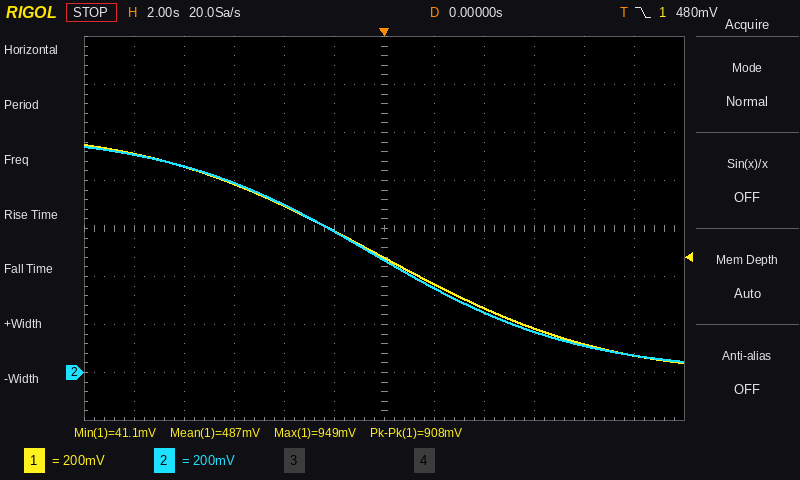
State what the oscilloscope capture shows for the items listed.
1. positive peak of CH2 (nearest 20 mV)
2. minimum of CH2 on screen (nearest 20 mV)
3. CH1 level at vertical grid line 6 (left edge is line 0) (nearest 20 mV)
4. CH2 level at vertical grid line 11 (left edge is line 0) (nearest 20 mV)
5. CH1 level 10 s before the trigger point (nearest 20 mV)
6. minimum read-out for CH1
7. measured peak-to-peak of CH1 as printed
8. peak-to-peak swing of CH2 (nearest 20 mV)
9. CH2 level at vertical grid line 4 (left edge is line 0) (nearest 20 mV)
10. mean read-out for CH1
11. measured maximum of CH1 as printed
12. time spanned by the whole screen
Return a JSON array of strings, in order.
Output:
["940 mV", "40 mV", "480 mV", "80 mV", "920 mV", "41.1 mV", "908 mV", "900 mV", "700 mV", "487 mV", "949 mV", "24 s"]
